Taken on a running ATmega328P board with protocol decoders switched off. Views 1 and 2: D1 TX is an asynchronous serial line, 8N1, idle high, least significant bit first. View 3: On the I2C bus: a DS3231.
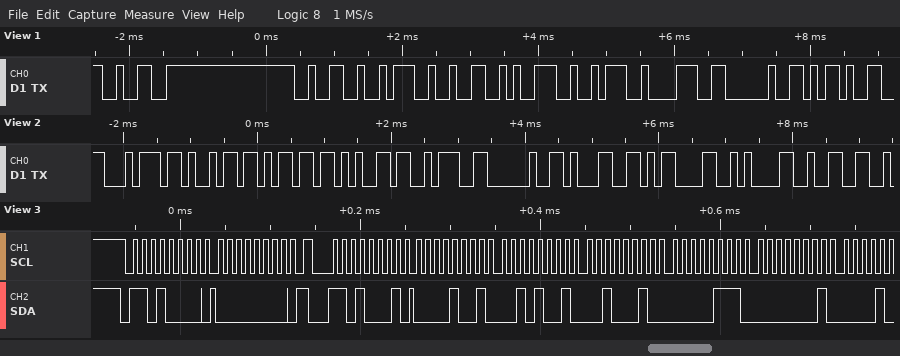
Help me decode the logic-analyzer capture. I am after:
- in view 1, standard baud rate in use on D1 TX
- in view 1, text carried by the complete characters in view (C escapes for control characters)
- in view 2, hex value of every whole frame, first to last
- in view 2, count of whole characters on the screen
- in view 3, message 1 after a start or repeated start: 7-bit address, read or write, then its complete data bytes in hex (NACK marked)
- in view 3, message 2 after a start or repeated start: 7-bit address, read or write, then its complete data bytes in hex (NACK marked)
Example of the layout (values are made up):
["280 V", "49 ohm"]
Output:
["9600 baud", "\"22:29:8 -\"", "0x74 0x69 0x6D 0x65 0x3A 0x20 0x31 0x0D 0x0A 0x32", "10", "0x68 write: 00", "0x68 read: 09 29 22 07 01"]
